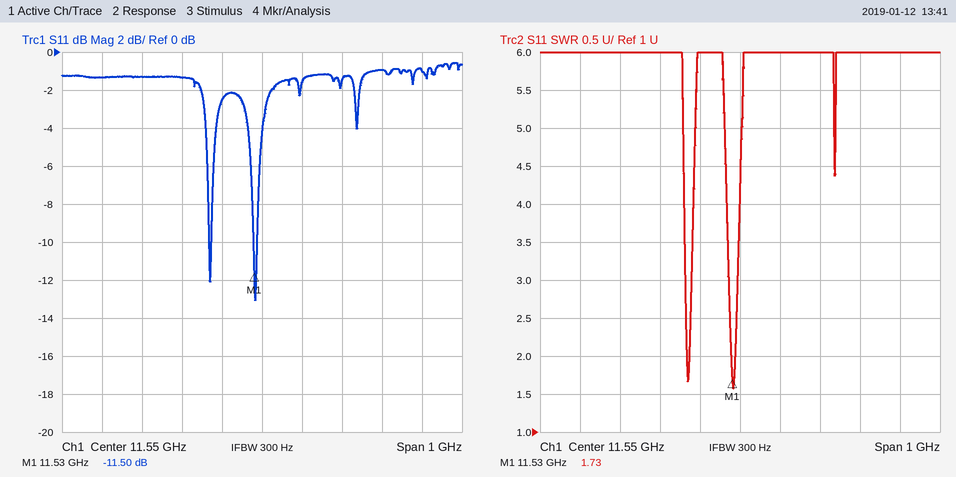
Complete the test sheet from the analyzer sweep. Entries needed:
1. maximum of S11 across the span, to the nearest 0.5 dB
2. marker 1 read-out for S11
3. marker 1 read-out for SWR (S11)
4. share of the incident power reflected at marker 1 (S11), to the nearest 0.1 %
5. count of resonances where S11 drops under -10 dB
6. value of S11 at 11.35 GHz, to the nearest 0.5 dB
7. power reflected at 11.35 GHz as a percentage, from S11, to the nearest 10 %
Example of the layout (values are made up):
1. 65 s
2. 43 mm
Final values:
1. -0.5 dB
2. -11.50 dB
3. 1.73
4. 7.1 %
5. 2
6. -1.5 dB
7. 70 %
